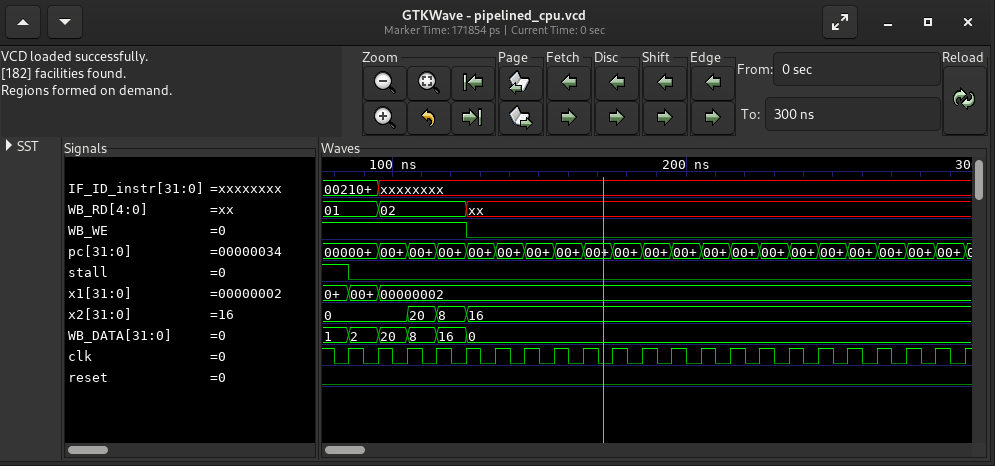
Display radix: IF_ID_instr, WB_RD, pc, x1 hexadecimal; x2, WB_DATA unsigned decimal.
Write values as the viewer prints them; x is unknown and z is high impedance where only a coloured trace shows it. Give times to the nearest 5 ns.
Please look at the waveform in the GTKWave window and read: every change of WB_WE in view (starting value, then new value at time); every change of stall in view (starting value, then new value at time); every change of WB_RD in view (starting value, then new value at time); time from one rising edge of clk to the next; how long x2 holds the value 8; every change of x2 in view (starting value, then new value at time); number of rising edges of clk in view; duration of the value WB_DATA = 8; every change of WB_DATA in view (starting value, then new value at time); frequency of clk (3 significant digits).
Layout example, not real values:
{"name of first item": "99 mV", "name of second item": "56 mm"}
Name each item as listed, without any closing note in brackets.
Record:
{"every change of WB_WE in view": "1, 0 at 125 ns", "every change of stall in view": "1, 0 at 85 ns", "every change of WB_RD in view": "01, 02 at 95 ns, xx at 125 ns", "time from one rising edge of clk to the next": "10 ns", "how long x2 holds the value 8": "10 ns", "every change of x2 in view": "0, 20 at 105 ns, 8 at 115 ns, 16 at 125 ns", "number of rising edges of clk in view": "22", "duration of the value WB_DATA = 8": "10 ns", "every change of WB_DATA in view": "1, 2 at 85 ns, 20 at 95 ns, 8 at 105 ns, 16 at 115 ns, 0 at 125 ns", "frequency of clk": "100 MHz"}
